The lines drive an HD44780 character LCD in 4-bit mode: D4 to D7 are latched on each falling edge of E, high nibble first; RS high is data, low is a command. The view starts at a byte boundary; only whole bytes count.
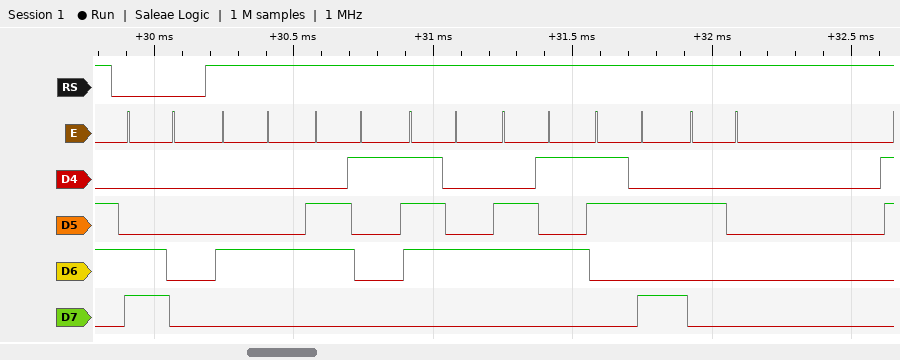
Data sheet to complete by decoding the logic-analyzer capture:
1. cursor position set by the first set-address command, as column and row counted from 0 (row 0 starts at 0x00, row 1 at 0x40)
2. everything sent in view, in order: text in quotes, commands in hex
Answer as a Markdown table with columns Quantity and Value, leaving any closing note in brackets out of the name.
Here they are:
| Quantity | Value |
|---|---|
| cursor position set by the first set-address command, as column and row counted from 0 | column 0, row 1 |
| everything sent in view, in order: text in quotes, commands in hex | 0xC0 "Date: " |
